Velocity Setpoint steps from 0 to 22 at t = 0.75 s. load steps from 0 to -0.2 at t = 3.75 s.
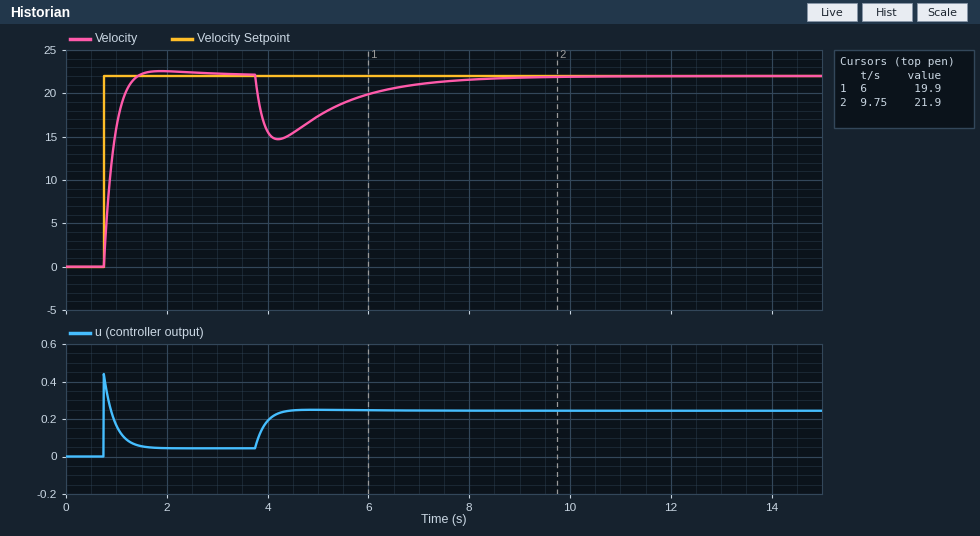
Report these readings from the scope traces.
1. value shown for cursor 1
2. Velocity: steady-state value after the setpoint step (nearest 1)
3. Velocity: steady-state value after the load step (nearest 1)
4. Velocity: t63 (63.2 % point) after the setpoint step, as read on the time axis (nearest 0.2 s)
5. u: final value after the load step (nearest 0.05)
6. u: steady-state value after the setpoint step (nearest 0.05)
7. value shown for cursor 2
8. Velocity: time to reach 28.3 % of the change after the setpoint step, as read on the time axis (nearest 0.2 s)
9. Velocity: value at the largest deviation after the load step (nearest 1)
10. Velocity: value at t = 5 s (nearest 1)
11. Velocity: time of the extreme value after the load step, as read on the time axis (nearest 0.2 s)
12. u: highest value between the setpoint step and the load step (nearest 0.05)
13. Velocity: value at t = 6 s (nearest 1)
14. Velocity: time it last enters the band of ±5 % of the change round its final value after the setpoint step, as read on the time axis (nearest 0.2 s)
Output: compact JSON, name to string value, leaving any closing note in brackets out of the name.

{"value shown for cursor 1": "19.9", "Velocity: steady-state value after the setpoint step": "22", "Velocity: steady-state value after the load step": "22", "Velocity: t63 (63.2 % point) after the setpoint step, as read on the time axis": "1.0 s", "u: final value after the load step": "0.25", "u: steady-state value after the setpoint step": "0.05", "value shown for cursor 2": "21.9", "Velocity: time to reach 28.3 % of the change after the setpoint step, as read on the time axis": "0.8 s", "Velocity: value at the largest deviation after the load step": "15", "Velocity: value at t = 5 s": "17", "Velocity: time of the extreme value after the load step, as read on the time axis": "4.2 s", "u: highest value between the setpoint step and the load step": "0.45", "Velocity: value at t = 6 s": "20", "Velocity: time it last enters the band of ±5 % of the change round its final value after the setpoint step, as read on the time axis": "1.2 s"}
